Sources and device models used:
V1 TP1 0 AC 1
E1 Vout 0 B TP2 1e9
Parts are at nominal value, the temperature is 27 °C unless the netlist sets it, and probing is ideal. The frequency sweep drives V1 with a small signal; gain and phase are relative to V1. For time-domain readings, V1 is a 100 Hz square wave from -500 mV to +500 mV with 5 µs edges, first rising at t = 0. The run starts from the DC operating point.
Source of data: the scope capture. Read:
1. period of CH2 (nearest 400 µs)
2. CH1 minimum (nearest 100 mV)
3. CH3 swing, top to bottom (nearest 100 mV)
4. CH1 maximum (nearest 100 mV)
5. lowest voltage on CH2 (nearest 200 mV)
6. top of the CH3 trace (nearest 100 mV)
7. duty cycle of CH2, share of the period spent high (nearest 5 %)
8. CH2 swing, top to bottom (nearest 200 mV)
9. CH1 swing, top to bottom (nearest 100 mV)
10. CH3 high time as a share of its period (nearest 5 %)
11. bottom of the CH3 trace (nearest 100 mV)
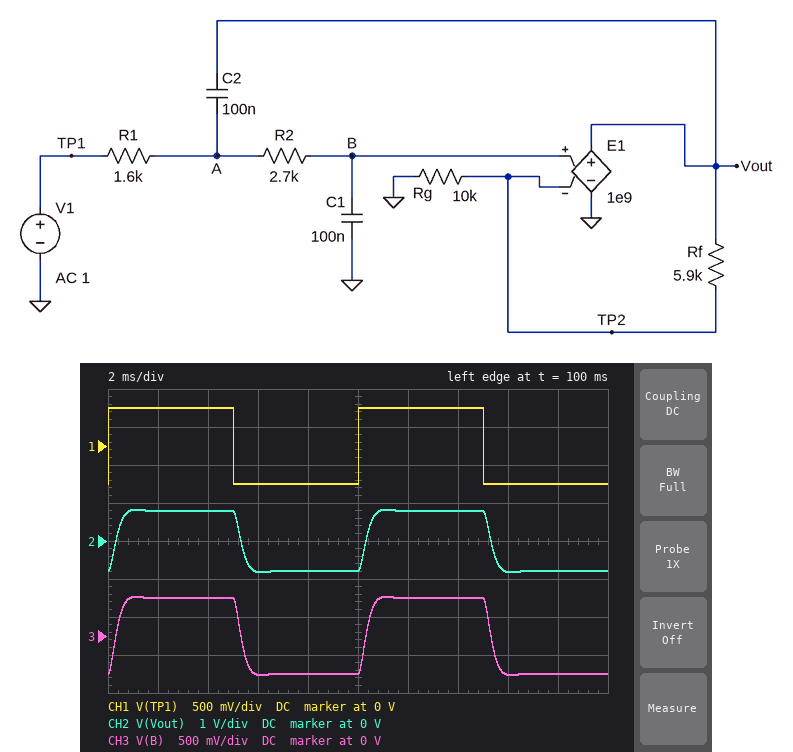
10.0 ms
-500 mV
1.0 V
500 mV
-800 mV
500 mV
50 %
1.6 V
1.0 V
50 %
-500 mV
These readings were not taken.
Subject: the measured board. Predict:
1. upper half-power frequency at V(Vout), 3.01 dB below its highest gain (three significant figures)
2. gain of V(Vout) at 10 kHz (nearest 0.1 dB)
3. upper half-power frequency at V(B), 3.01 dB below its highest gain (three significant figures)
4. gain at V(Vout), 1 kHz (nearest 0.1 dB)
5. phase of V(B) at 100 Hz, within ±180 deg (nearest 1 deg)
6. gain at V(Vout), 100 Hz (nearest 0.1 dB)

659 Hz
-40.6 dB
659 Hz
-2.9 dB
-12 deg
4.0 dB
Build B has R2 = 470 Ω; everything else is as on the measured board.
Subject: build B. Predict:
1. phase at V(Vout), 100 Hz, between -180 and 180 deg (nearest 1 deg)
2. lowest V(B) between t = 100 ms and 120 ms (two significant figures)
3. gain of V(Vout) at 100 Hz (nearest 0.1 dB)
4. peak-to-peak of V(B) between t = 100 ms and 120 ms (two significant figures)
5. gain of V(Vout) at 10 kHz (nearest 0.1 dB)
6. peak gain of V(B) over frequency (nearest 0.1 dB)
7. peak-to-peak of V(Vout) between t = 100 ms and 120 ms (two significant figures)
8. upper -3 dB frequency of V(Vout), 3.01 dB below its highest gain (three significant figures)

-4 deg
-570 mV
4.0 dB
1.1 V
-25.4 dB
0.1 dB
1.8 V
1.96 kHz
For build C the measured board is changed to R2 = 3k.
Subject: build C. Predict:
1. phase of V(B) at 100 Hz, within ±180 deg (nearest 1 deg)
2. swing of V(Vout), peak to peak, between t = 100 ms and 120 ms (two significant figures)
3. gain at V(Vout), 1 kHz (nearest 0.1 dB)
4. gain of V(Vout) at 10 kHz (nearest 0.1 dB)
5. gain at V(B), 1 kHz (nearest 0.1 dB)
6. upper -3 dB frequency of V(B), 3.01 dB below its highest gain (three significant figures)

-13 deg
1.6 V
-3.8 dB
-41.5 dB
-7.8 dB
600 Hz
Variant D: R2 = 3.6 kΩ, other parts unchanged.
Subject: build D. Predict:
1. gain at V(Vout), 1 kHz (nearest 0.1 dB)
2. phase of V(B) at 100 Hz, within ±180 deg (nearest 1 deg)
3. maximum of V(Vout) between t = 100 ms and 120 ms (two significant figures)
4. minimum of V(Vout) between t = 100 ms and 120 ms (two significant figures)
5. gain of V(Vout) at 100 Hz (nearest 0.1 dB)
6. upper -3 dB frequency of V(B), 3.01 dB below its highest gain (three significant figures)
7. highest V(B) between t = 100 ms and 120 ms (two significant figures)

-5.4 dB
-15 deg
800 mV
-800 mV
3.9 dB
505 Hz
500 mV
